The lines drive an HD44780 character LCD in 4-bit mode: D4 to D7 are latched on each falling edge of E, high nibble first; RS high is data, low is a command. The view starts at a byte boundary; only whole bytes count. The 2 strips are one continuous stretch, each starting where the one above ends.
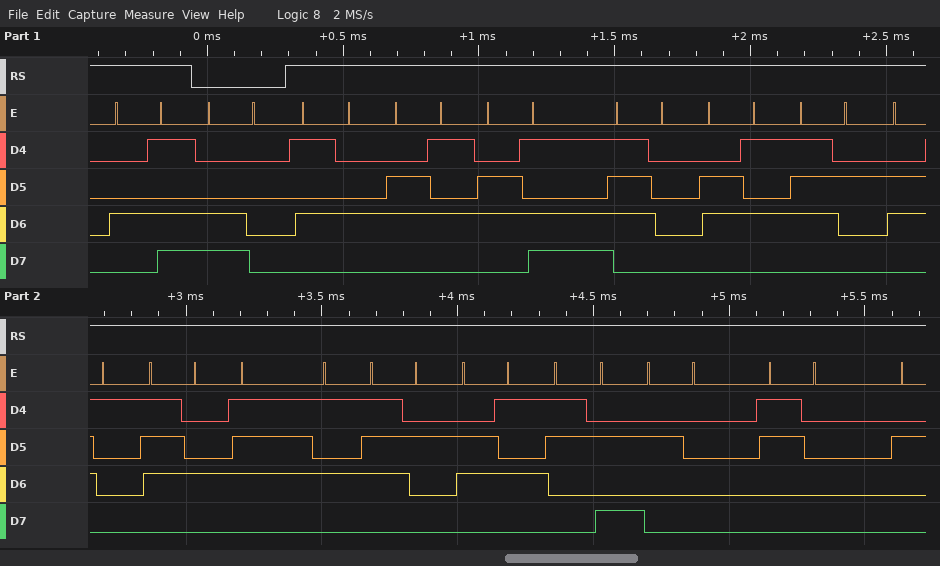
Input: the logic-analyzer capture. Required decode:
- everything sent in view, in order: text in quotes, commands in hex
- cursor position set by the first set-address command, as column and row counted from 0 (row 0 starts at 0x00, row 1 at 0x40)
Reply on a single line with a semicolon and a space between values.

"M" 0xC0 "Temperature: 0"; column 0, row 1
